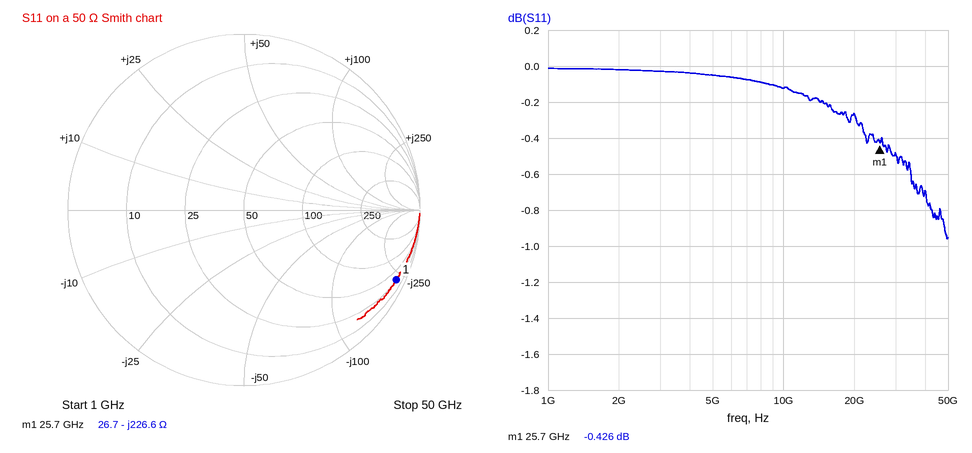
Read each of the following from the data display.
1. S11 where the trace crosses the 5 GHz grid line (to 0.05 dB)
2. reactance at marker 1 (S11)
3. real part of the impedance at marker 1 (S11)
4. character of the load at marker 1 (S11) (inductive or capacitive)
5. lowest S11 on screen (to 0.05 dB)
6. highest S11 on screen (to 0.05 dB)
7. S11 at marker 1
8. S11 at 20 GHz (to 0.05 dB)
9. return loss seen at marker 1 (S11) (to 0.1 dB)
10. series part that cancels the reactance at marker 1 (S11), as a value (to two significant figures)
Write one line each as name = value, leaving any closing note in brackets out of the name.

S11 where the trace crosses the 5 GHz grid line = -0.05 dB
reactance at marker 1 = -226.6 Ω
real part of the impedance at marker 1 = 26.7 Ω
character of the load at marker 1 (S11) = capacitive
lowest S11 on screen = -0.95 dB
highest S11 on screen = 0.00 dB
S11 at marker 1 = -0.426 dB
S11 at 20 GHz = -0.25 dB
return loss seen at marker 1 (S11) = 0.4 dB
series part that cancels the reactance at marker 1 (S11), as a value = 1.4 nH
